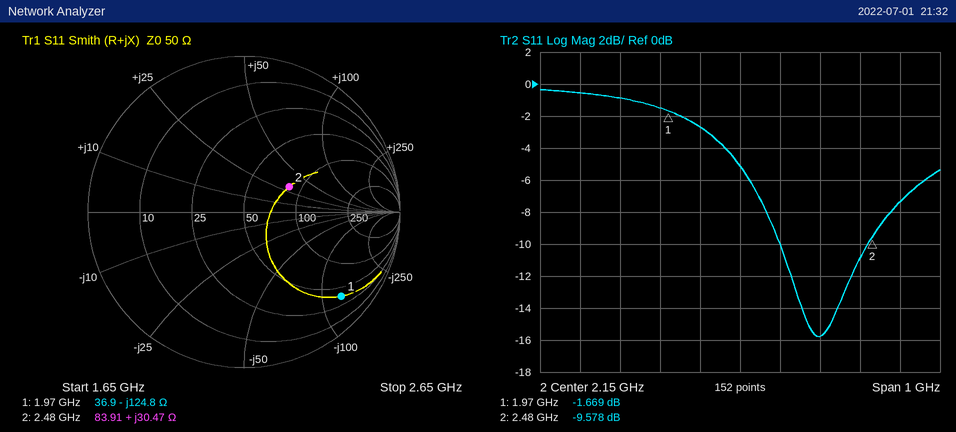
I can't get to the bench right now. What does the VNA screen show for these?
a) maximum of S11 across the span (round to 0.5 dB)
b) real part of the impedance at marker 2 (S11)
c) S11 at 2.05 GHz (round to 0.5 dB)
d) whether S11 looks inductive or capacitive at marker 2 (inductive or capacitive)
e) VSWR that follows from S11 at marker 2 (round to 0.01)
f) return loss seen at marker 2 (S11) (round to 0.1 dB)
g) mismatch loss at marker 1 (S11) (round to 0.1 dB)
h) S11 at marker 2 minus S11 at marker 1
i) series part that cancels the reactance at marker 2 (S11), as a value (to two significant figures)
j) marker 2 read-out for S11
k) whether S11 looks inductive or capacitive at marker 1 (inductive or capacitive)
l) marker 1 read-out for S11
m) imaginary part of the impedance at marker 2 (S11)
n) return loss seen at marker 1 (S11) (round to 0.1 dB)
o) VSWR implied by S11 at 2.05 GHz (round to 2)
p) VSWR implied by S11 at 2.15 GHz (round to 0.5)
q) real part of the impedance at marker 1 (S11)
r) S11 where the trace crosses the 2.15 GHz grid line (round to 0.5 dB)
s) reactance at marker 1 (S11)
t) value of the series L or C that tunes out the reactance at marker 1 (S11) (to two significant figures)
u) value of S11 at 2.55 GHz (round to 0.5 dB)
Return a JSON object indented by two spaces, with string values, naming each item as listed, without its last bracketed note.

{
  "maximum of S11 across the span": "-0.5 dB",
  "real part of the impedance at marker 2": "83.91 Ω",
  "S11 at 2.05 GHz": "-2.5 dB",
  "whether S11 looks inductive or capacitive at marker 2": "inductive",
  "VSWR that follows from S11 at marker 2": "1.99",
  "return loss seen at marker 2 (S11)": "9.6 dB",
  "mismatch loss at marker 1 (S11)": "5.0 dB",
  "S11 at marker 2 minus S11 at marker 1": "-7.909 dB",
  "series part that cancels the reactance at marker 2 (S11), as a value": "2.1 pF",
  "marker 2 read-out for S11": "-9.578 dB",
  "whether S11 looks inductive or capacitive at marker 1": "capacitive",
  "marker 1 read-out for S11": "-1.669 dB",
  "imaginary part of the impedance at marker 2": "+30.47 Ω",
  "return loss seen at marker 1 (S11)": "1.7 dB",
  "VSWR implied by S11 at 2.05 GHz": "6",
  "VSWR implied by S11 at 2.15 GHz": "3.5",
  "real part of the impedance at marker 1": "36.9 Ω",
  "S11 where the trace crosses the 2.15 GHz grid line": "-5.0 dB",
  "reactance at marker 1": "-124.8 Ω",
  "value of the series L or C that tunes out the reactance at marker 1 (S11)": "10 nH",
  "value of S11 at 2.55 GHz": "-7.5 dB"
}
